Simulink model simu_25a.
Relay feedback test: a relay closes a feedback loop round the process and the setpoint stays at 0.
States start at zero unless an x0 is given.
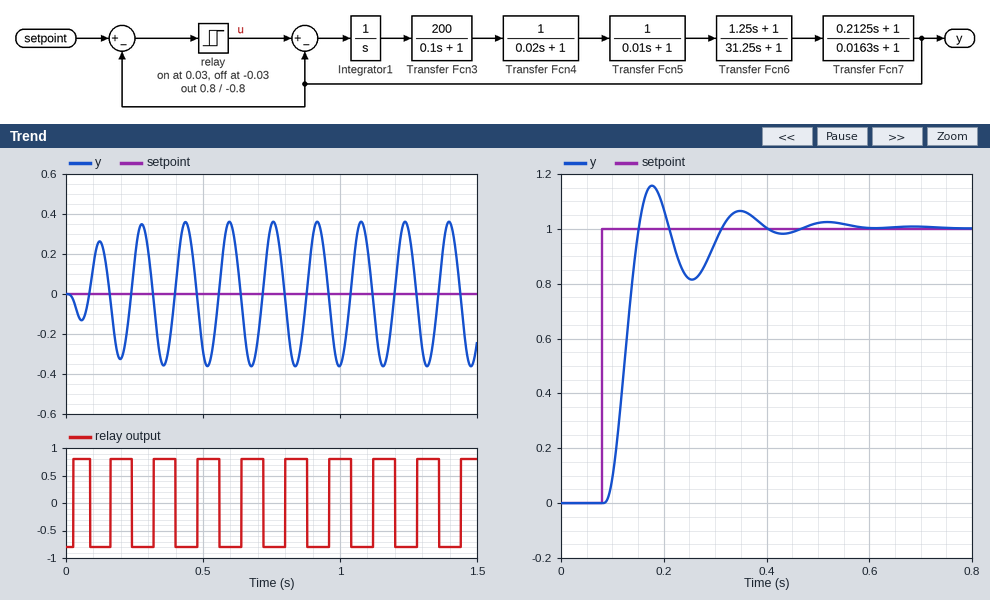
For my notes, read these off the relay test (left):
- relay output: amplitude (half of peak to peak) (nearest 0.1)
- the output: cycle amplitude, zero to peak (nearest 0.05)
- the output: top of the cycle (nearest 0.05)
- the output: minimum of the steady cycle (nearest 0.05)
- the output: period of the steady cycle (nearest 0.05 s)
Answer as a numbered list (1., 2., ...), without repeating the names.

1. 0.8
2. 0.35
3. 0.35
4. -0.35
5. 0.15 s
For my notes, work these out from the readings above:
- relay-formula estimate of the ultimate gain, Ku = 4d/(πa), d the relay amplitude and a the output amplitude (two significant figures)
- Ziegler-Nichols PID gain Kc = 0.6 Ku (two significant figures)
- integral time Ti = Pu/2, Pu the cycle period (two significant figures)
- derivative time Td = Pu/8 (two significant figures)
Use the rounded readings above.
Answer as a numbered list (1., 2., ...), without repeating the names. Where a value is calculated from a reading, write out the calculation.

1. 4 × 0.8 / (π × 0.35) = 2.9
2. 0.6 × 2.9 = 1.7
3. 0.15 / 2 = 0.075 s
4. 0.15 / 8 = 0.019 s
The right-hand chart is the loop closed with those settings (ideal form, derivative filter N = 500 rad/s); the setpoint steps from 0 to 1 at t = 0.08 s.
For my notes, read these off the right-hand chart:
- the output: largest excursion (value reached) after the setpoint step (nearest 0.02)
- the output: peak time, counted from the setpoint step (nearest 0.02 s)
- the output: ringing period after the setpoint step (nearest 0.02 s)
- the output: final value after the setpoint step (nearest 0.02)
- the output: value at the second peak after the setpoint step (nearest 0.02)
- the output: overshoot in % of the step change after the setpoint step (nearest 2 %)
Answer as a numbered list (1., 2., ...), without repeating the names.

1. 1.16
2. 0.10 s
3. 0.18 s
4. 1.00
5. 1.06
6. 16 %
